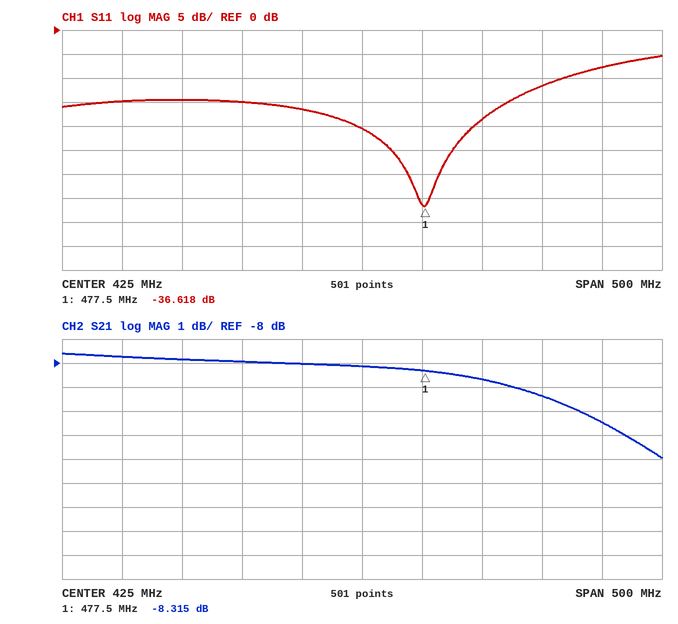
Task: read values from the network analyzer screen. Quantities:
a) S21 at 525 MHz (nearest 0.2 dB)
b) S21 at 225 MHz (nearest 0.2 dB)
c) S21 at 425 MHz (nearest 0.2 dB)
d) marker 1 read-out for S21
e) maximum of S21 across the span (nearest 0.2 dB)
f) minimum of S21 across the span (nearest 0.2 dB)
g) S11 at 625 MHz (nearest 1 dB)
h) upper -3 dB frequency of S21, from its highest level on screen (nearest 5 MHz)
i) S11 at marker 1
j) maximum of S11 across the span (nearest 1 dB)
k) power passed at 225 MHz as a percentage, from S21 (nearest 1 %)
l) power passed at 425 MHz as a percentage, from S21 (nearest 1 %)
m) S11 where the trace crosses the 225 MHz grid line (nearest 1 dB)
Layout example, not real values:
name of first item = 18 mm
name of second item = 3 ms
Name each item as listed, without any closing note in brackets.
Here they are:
S21 at 525 MHz = -8.6 dB
S21 at 225 MHz = -7.8 dB
S21 at 425 MHz = -8.2 dB
marker 1 read-out for S21 = -8.315 dB
maximum of S21 across the span = -7.6 dB
minimum of S21 across the span = -12.0 dB
S11 at 625 MHz = -8 dB
upper -3 dB frequency of S21, from its highest level on screen = 630 MHz
S11 at marker 1 = -36.618 dB
maximum of S11 across the span = -5 dB
power passed at 225 MHz as a percentage, from S21 = 17 %
power passed at 425 MHz as a percentage, from S21 = 15 %
S11 where the trace crosses the 225 MHz grid line = -15 dB
